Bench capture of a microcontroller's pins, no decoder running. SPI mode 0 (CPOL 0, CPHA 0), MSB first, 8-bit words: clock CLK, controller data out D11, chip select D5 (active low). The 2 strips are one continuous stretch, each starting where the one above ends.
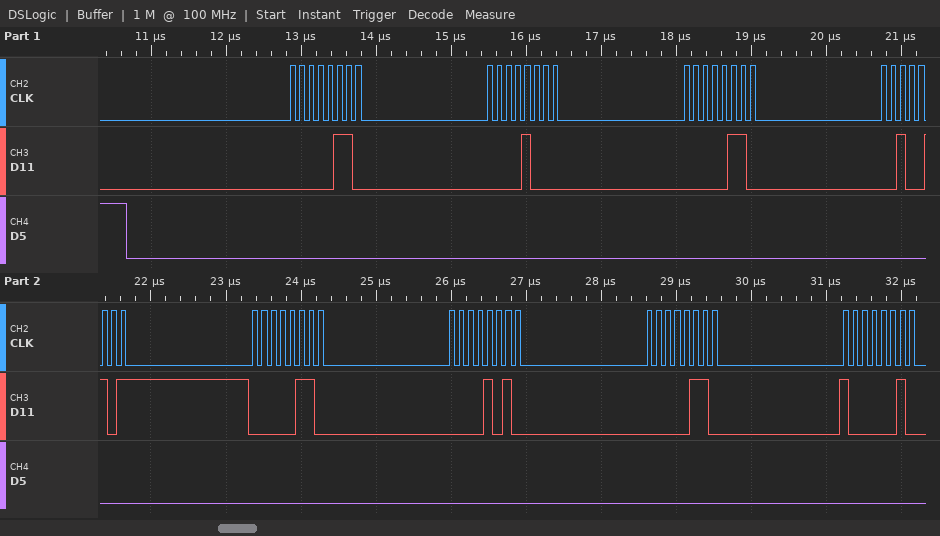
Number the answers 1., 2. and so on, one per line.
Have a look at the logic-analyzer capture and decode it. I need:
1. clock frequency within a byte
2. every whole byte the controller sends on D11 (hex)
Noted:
1. 8 MHz
2. 0x06 0x08 0x06 0x25 0x06 0x0A 0x06 0x82
